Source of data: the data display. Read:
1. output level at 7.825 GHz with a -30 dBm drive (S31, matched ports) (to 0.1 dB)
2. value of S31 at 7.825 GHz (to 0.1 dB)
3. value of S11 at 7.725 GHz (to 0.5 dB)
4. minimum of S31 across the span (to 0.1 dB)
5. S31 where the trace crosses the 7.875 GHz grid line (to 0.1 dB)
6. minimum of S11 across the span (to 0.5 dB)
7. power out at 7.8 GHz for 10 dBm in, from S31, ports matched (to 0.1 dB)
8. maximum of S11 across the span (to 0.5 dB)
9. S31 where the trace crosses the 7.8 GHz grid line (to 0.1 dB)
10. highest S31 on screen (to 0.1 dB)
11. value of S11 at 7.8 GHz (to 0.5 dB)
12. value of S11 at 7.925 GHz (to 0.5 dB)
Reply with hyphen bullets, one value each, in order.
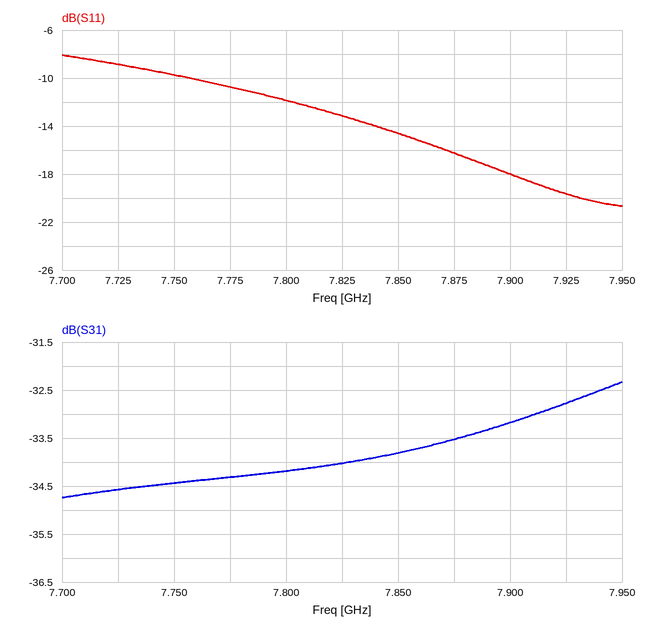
- -64.0 dBm
- -34.0 dB
- -9.0 dB
- -34.7 dB
- -33.5 dB
- -20.5 dB
- -24.2 dBm
- -8.0 dB
- -34.2 dB
- -32.3 dB
- -12.0 dB
- -19.5 dB
